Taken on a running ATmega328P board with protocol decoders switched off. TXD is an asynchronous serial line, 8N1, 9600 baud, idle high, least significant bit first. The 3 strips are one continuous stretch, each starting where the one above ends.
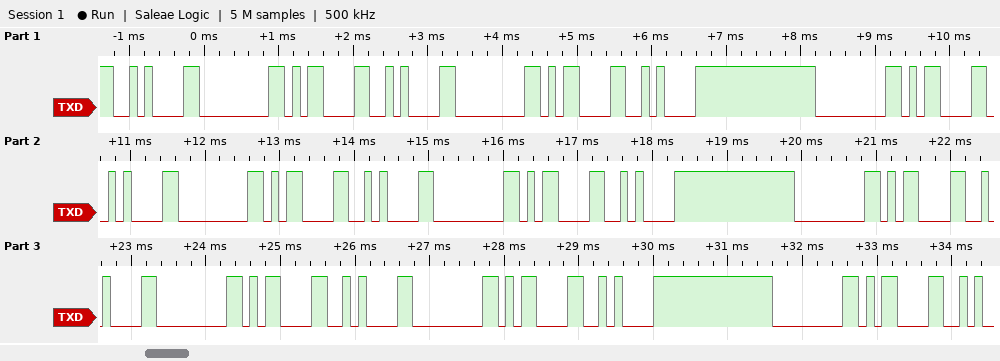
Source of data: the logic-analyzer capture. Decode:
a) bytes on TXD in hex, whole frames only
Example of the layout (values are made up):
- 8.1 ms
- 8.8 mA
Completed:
- 0x0A 0x00 0x0D 0x0A 0x00 0x0D 0x0A 0x00 0x0D 0x0A 0x00 0x0D 0x0A 0x00 0x0D 0x0A 0x00 0x0D 0x0A 0x00 0x0D 0x0A 0x00 0x0D 0x0A 0x00 0x0D
